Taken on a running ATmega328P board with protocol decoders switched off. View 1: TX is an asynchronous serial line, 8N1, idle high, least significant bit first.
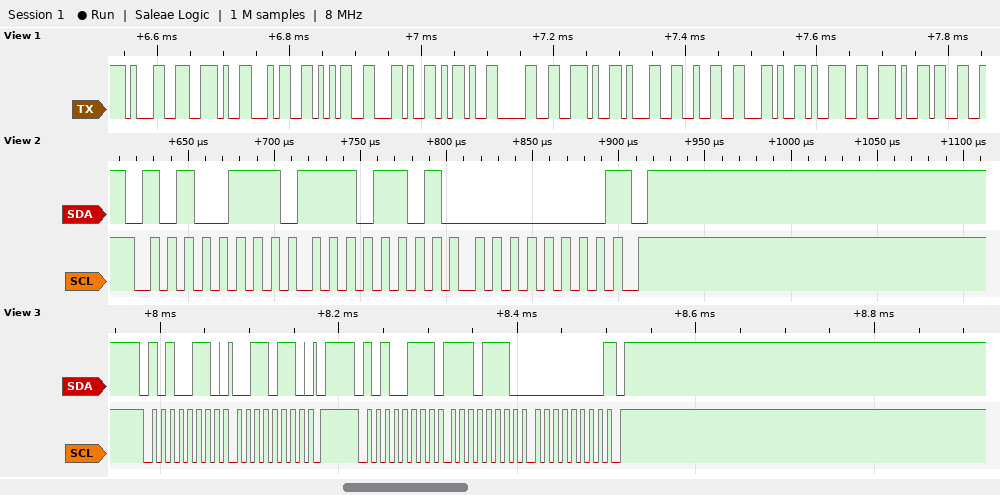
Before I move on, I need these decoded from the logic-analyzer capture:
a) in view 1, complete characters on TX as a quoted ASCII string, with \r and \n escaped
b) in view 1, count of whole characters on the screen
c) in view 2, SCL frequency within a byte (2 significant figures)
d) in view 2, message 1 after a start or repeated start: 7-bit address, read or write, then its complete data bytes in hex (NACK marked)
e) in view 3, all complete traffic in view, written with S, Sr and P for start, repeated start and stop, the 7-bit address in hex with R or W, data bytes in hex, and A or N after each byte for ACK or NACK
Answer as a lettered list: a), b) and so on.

a) "1.45,-0.12,9.3"
b) 14
c) 100 kHz
d) 0x53 read: ED 00 NACK
e) S 53W A 36 A P S 53R A EE A 00 N P
